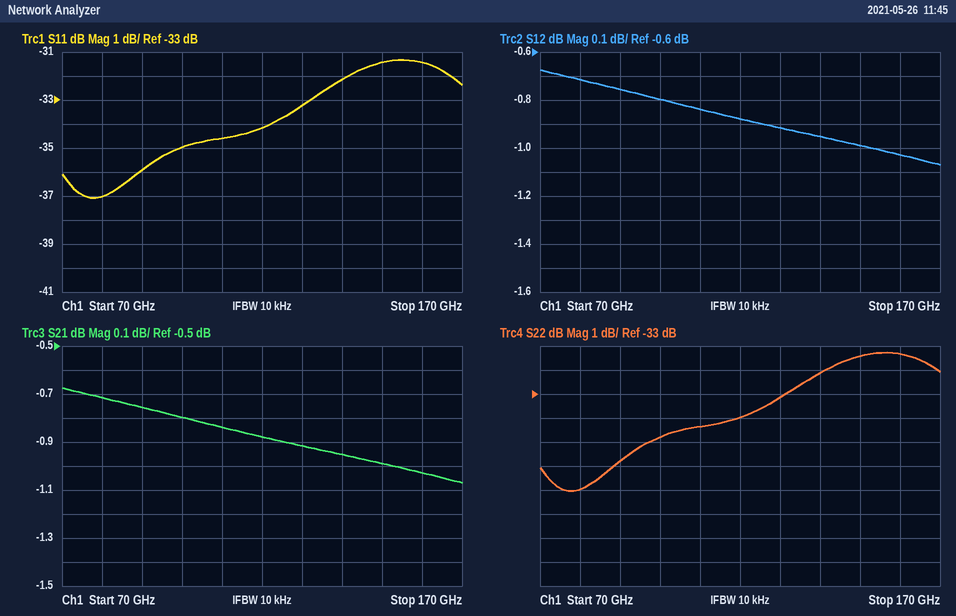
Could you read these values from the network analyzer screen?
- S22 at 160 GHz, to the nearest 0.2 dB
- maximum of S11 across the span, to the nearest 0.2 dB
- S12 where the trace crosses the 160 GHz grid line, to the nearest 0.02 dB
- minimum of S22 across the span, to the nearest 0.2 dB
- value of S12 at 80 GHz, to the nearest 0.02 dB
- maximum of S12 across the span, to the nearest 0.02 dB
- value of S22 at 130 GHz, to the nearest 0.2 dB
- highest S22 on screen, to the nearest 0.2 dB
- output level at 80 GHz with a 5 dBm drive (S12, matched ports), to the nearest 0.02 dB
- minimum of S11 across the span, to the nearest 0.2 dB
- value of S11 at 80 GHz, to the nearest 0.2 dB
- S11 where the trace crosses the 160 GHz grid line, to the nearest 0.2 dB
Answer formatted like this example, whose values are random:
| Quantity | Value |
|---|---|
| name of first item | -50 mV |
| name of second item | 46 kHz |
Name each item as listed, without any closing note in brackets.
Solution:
| Quantity | Value |
|---|---|
| S22 at 160 GHz, to the nearest 0.2 dB | -31.4 dB |
| maximum of S11 across the span, to the nearest 0.2 dB | -31.4 dB |
| S12 where the trace crosses the 160 GHz grid line, to the nearest 0.02 dB | -1.02 dB |
| minimum of S22 across the span, to the nearest 0.2 dB | -37.0 dB |
| value of S12 at 80 GHz, to the nearest 0.02 dB | -0.72 dB |
| maximum of S12 across the span, to the nearest 0.02 dB | -0.68 dB |
| value of S22 at 130 GHz, to the nearest 0.2 dB | -33.2 dB |
| highest S22 on screen, to the nearest 0.2 dB | -31.2 dB |
| output level at 80 GHz with a 5 dBm drive (S12, matched ports), to the nearest 0.02 dB | 4.28 dBm |
| minimum of S11 across the span, to the nearest 0.2 dB | -37.0 dB |
| value of S11 at 80 GHz, to the nearest 0.2 dB | -37.0 dB |
| S11 where the trace crosses the 160 GHz grid line, to the nearest 0.2 dB | -31.4 dB |
